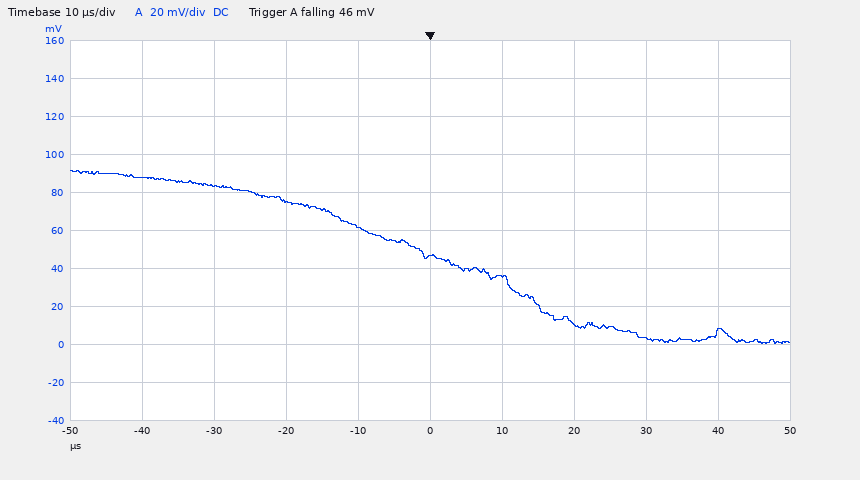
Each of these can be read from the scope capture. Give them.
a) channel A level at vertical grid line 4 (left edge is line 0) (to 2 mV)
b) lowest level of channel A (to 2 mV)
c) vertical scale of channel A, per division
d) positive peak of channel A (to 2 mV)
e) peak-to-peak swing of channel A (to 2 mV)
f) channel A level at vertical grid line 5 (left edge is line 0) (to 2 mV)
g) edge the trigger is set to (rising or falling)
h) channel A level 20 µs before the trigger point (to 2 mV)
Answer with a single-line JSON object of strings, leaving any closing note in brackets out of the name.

{"channel A level at vertical grid line 4 (left edge is line 0)": "62 mV", "lowest level of channel A": "0 mV", "vertical scale of channel A, per division": "20 mV", "positive peak of channel A": "92 mV", "peak-to-peak swing of channel A": "92 mV", "channel A level at vertical grid line 5 (left edge is line 0)": "46 mV", "edge the trigger is set to": "falling", "channel A level 20 µs before the trigger point": "76 mV"}
